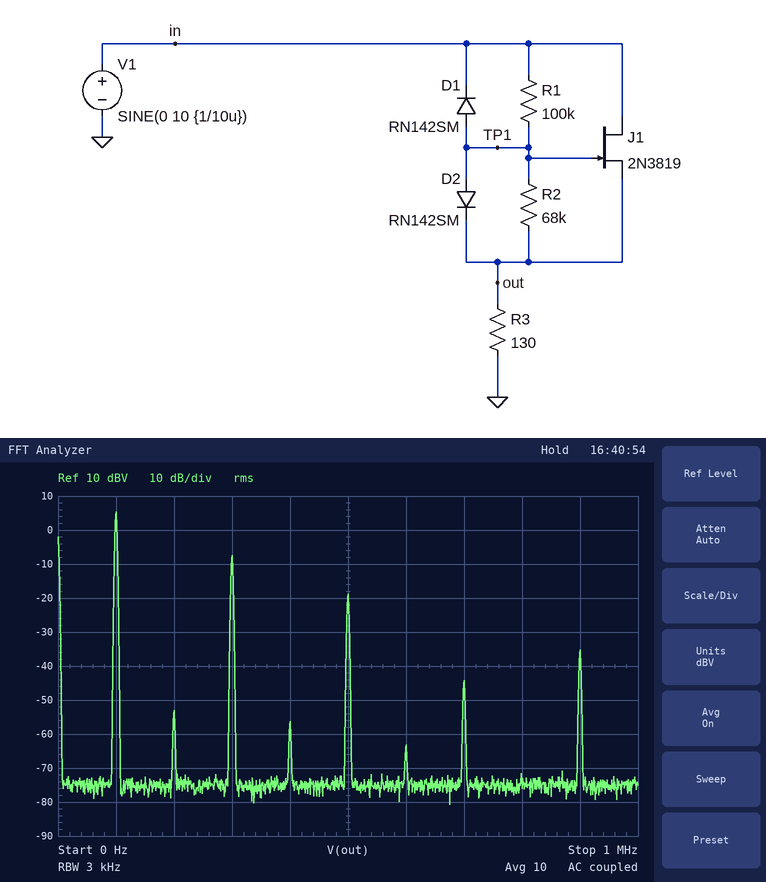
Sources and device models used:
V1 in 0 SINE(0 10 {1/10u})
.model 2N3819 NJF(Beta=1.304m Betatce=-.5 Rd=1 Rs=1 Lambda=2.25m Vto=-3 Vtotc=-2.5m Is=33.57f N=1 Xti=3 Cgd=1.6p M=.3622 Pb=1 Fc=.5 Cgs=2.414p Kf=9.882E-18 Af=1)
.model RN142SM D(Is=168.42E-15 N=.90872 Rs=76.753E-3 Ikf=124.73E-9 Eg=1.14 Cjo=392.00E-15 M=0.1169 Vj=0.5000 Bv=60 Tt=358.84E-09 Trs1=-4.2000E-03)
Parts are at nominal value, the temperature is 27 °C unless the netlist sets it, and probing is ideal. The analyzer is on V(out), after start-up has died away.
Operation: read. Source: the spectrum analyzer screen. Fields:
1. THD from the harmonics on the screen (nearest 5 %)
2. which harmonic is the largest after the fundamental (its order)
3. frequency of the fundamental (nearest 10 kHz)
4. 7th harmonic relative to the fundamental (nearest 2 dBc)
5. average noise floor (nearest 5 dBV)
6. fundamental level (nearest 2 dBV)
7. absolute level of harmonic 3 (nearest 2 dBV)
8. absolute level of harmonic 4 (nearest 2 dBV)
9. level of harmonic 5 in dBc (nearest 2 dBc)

25 %
3
100 kHz
-50 dBc
-75 dBV
6 dBV
-8 dBV
-56 dBV
-24 dBc
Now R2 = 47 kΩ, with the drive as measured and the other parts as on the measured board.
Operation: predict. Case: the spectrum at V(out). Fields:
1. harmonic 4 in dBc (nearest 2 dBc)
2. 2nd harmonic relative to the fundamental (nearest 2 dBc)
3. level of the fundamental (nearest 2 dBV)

-56 dBc
-52 dBc
6 dBV
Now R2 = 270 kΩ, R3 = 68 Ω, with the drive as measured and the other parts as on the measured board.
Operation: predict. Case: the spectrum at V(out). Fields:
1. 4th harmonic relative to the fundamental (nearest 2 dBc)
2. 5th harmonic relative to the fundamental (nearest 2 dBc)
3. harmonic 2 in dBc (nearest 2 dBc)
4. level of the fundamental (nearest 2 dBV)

-48 dBc
-20 dBc
-48 dBc
0 dBV
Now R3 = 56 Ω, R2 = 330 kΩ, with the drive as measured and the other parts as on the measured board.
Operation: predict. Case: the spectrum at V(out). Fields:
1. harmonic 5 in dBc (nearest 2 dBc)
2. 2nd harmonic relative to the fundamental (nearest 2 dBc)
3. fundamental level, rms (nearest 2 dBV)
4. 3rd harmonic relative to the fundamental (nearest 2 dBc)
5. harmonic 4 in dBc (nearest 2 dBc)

-20 dBc
-46 dBc
-2 dBV
-12 dBc
-44 dBc
